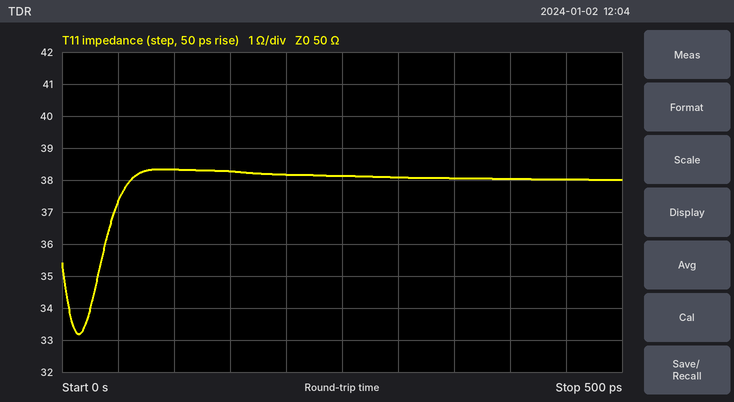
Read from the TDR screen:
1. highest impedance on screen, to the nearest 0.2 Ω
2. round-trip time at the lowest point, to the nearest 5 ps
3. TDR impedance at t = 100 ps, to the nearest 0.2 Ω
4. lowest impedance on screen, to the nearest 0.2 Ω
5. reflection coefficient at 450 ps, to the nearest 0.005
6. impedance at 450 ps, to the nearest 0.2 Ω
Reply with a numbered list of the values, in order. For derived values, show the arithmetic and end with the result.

1. 38.4 Ω
2. 15 ps
3. 38.4 Ω
4. 33.2 Ω
5. (38 − 50)/(38 + 50) ≈ -0.136, so -0.135 to the nearest 0.005
6. 38.0 Ω
